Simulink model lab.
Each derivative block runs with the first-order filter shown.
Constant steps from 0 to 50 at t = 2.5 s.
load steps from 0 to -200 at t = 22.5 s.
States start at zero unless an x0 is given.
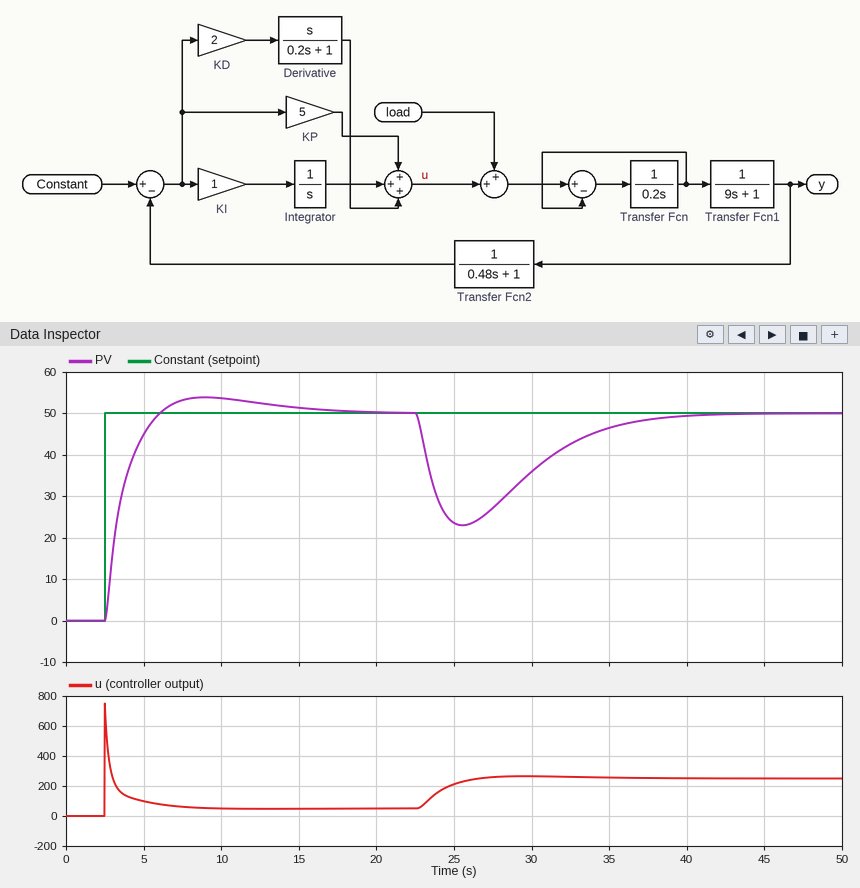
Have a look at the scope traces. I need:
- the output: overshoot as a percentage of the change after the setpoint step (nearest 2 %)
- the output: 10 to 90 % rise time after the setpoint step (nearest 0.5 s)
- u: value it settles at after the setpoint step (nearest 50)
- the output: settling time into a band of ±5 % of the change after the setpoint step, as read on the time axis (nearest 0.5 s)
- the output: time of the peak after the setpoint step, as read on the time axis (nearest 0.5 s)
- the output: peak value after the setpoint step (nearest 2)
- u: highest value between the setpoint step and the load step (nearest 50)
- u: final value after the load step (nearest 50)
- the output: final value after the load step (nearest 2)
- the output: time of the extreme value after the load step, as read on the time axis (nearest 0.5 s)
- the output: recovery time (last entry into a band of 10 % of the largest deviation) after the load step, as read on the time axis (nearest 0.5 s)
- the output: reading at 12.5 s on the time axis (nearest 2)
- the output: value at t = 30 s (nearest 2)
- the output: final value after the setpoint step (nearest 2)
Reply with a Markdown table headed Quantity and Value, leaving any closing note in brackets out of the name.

| Quantity | Value |
|---|---|
| the output: overshoot as a percentage of the change after the setpoint step | 8 % |
| the output: 10 to 90 % rise time after the setpoint step | 2.5 s |
| u: value it settles at after the setpoint step | 50 |
| the output: settling time into a band of ±5 % of the change after the setpoint step, as read on the time axis | 12.5 s |
| the output: time of the peak after the setpoint step, as read on the time axis | 9.0 s |
| the output: peak value after the setpoint step | 54 |
| u: highest value between the setpoint step and the load step | 750 |
| u: final value after the load step | 250 |
| the output: final value after the load step | 50 |
| the output: time of the extreme value after the load step, as read on the time axis | 25.5 s |
| the output: recovery time (last entry into a band of 10 % of the largest deviation) after the load step, as read on the time axis | 36.0 s |
| the output: reading at 12.5 s on the time axis | 52 |
| the output: value at t = 30 s | 36 |
| the output: final value after the setpoint step | 50 |
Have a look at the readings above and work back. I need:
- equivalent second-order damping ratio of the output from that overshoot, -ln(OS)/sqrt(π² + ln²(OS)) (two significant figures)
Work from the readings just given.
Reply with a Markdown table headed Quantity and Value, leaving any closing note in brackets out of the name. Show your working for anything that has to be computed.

| Quantity | Value |
|---|---|
| equivalent second-order damping ratio of the output from that overshoot, -ln(OS)/sqrt(π² + ln²(OS)) | ln(0.08) = -2.526; 2.526 / sqrt(9.870 + 6.379) = 0.63 |
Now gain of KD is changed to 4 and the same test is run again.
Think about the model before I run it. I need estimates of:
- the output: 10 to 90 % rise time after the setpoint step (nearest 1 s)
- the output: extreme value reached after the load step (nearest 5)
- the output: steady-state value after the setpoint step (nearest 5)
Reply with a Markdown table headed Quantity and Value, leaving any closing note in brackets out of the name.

| Quantity | Value |
|---|---|
| the output: 10 to 90 % rise time after the setpoint step | 3 s |
| the output: extreme value reached after the load step | 25 |
| the output: steady-state value after the setpoint step | 50 |
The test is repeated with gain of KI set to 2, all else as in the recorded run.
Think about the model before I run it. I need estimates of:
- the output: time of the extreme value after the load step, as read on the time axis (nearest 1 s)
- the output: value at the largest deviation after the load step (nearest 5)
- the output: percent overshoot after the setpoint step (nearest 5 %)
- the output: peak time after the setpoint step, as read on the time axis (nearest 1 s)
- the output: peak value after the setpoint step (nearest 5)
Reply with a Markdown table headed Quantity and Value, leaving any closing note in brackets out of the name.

| Quantity | Value |
|---|---|
| the output: time of the extreme value after the load step, as read on the time axis | 25 s |
| the output: value at the largest deviation after the load step | 25 |
| the output: percent overshoot after the setpoint step | 20 % |
| the output: peak time after the setpoint step, as read on the time axis | 7 s |
| the output: peak value after the setpoint step | 60 |
